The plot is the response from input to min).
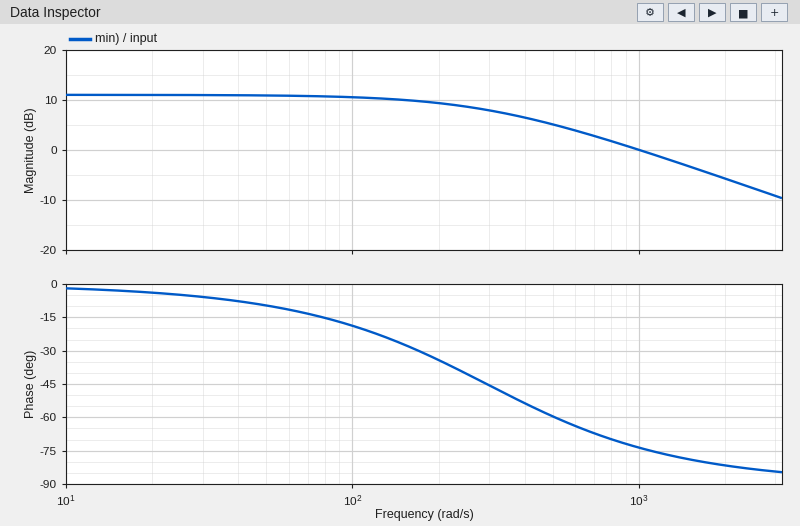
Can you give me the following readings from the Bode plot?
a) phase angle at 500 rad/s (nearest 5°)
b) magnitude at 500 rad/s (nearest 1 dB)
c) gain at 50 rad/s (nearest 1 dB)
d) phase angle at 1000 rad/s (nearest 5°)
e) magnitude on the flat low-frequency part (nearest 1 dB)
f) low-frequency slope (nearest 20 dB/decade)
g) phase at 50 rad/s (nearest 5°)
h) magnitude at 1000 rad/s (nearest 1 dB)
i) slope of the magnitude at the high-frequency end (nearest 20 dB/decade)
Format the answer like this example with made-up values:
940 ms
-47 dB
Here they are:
-60°
5 dB
11 dB
-75°
11 dB
0 dB/decade
-10°
0 dB
-20 dB/decade
